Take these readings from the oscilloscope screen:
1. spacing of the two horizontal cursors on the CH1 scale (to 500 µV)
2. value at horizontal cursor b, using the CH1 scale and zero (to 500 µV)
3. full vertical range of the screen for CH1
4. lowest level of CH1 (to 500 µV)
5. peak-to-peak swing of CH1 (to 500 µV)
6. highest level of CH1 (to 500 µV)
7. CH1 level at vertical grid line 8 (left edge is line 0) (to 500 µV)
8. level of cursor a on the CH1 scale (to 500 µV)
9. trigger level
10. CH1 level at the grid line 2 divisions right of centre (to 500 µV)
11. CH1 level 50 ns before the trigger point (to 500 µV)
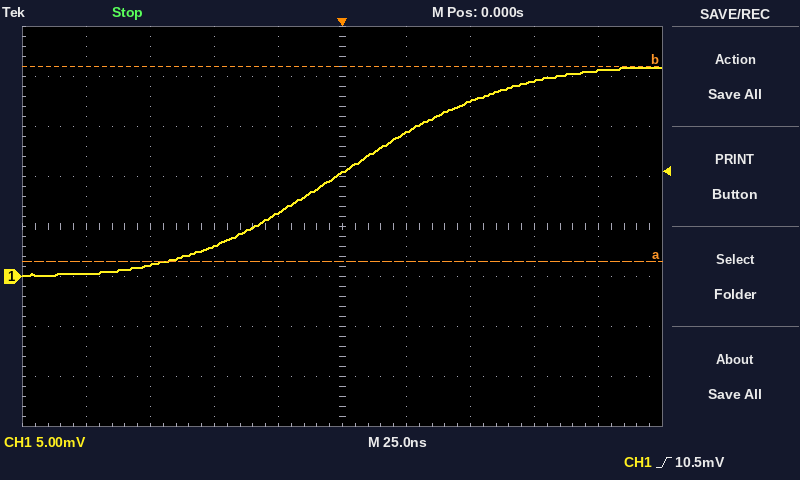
19.5 mV
21.0 mV
40 mV
0.0 mV
21.0 mV
21.0 mV
19.5 mV
1.5 mV
10.5 mV
17.5 mV
3.0 mV
